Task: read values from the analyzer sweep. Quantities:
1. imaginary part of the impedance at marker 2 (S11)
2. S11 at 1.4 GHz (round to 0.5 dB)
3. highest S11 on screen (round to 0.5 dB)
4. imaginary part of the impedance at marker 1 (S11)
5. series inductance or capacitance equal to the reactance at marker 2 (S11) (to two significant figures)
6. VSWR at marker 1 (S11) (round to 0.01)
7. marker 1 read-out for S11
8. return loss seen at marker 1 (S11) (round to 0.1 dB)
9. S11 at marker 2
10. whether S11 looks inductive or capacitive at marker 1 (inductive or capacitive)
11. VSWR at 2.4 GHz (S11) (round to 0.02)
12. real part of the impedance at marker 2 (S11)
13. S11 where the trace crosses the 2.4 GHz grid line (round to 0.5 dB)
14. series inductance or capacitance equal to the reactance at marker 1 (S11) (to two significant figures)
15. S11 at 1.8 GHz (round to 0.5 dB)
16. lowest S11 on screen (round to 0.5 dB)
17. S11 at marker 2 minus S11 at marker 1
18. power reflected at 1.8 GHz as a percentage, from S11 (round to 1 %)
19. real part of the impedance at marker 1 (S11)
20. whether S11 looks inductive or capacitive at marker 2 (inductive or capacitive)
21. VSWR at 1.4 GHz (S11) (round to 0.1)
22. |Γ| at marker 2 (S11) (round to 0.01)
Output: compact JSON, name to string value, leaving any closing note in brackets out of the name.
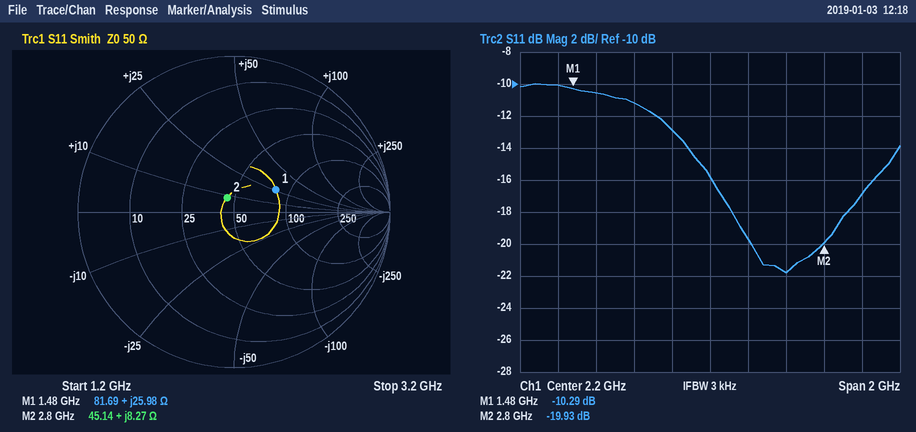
{"imaginary part of the impedance at marker 2": "+8.27 Ω", "S11 at 1.4 GHz": "-10.0 dB", "highest S11 on screen": "-10.0 dB", "imaginary part of the impedance at marker 1": "+25.98 Ω", "series inductance or capacitance equal to the reactance at marker 2 (S11)": "470 pH", "VSWR at marker 1 (S11)": "1.88", "marker 1 read-out for S11": "-10.29 dB", "return loss seen at marker 1 (S11)": "10.3 dB", "S11 at marker 2": "-19.93 dB", "whether S11 looks inductive or capacitive at marker 1": "inductive", "VSWR at 2.4 GHz (S11)": "1.24", "real part of the impedance at marker 2": "45.14 Ω", "S11 where the trace crosses the 2.4 GHz grid line": "-19.5 dB", "series inductance or capacitance equal to the reactance at marker 1 (S11)": "2.8 nH", "S11 at 1.8 GHz": "-11.0 dB", "lowest S11 on screen": "-22.0 dB", "S11 at marker 2 minus S11 at marker 1": "-9.64 dB", "power reflected at 1.8 GHz as a percentage, from S11": "8 %", "real part of the impedance at marker 1": "81.69 Ω", "whether S11 looks inductive or capacitive at marker 2": "inductive", "VSWR at 1.4 GHz (S11)": "1.9", "|Γ| at marker 2 (S11)": "0.10"}
